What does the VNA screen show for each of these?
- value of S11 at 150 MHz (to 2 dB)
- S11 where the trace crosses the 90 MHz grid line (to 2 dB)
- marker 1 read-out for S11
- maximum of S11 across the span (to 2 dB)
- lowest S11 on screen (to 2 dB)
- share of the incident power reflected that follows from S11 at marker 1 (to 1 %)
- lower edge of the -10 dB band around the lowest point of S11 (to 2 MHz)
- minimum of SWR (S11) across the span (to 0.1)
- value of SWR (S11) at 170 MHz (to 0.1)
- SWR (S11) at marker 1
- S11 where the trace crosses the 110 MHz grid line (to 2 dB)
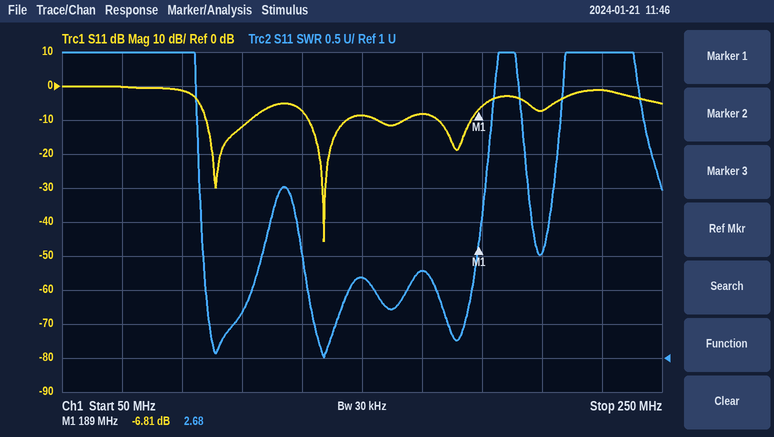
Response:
-8 dB
-2 dB
-6.81 dB
0 dB
-46 dB
21 %
132 MHz
1.0
2.3
2.68
-12 dB
